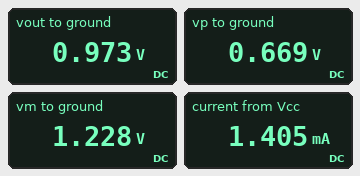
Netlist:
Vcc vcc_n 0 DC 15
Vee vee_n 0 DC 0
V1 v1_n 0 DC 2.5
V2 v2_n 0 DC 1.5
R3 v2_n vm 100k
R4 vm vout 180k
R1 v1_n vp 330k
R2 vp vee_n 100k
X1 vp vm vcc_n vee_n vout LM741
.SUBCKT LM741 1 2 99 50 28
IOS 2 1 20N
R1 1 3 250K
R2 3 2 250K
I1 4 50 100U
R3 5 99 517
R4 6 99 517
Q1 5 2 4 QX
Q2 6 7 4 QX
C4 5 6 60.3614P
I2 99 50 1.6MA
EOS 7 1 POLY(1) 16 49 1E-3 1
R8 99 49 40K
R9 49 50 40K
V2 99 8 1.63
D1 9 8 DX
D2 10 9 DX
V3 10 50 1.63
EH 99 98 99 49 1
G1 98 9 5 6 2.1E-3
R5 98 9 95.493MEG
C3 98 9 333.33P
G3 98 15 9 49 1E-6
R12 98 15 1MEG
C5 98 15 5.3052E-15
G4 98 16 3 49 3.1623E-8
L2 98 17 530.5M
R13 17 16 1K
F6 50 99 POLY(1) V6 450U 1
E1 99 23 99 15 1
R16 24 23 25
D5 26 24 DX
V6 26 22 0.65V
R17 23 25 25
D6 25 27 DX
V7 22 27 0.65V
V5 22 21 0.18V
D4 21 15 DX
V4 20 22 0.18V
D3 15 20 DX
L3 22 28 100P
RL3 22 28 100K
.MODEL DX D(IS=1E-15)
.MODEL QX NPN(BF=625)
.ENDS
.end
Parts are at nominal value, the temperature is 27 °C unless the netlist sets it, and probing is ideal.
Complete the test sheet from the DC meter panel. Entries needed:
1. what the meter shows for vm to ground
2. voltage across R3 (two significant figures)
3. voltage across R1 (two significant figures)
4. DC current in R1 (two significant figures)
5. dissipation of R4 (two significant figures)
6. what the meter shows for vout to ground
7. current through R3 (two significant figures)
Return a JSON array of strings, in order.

["1.228 V", "270 mV", "1.8 V", "5.5 µA", "360 nW", "0.973 V", "2.7 µA"]
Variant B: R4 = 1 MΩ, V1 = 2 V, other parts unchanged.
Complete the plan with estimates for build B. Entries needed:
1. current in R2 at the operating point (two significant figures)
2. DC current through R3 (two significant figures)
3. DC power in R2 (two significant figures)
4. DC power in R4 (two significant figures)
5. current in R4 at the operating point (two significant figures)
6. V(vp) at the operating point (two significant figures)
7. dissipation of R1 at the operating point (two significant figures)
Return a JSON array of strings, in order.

["5.8 µA", "2.0 µA", "3.3 µW", "110 nW", "330 nA", "580 mV", "6.1 µW"]
